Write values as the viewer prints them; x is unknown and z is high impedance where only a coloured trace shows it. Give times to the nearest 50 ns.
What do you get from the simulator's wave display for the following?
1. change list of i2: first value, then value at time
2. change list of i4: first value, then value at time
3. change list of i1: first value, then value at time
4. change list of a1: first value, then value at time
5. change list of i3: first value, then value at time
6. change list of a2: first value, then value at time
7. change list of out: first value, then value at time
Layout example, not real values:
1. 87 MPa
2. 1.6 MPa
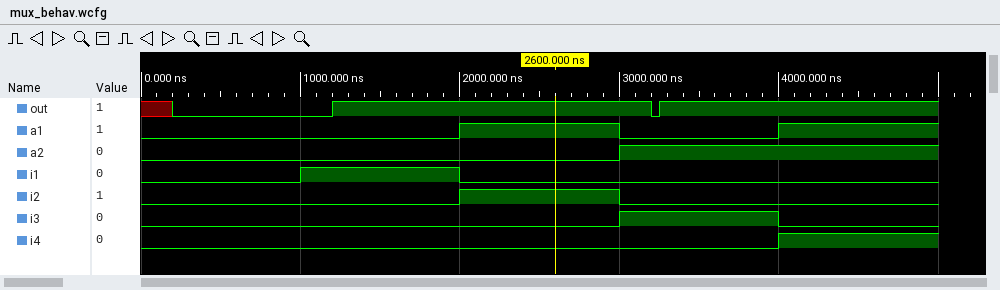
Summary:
1. 0, 1 at 2000 ns, 0 at 3000 ns
2. 0, 1 at 4000 ns
3. 0, 1 at 1000 ns, 0 at 2000 ns
4. 0, 1 at 2000 ns, 0 at 3000 ns, 1 at 4000 ns
5. 0, 1 at 3000 ns, 0 at 4000 ns
6. 0, 1 at 3000 ns
7. x, 0 at 200 ns, 1 at 1200 ns, 0 at 3200 ns, 1 at 3250 ns
